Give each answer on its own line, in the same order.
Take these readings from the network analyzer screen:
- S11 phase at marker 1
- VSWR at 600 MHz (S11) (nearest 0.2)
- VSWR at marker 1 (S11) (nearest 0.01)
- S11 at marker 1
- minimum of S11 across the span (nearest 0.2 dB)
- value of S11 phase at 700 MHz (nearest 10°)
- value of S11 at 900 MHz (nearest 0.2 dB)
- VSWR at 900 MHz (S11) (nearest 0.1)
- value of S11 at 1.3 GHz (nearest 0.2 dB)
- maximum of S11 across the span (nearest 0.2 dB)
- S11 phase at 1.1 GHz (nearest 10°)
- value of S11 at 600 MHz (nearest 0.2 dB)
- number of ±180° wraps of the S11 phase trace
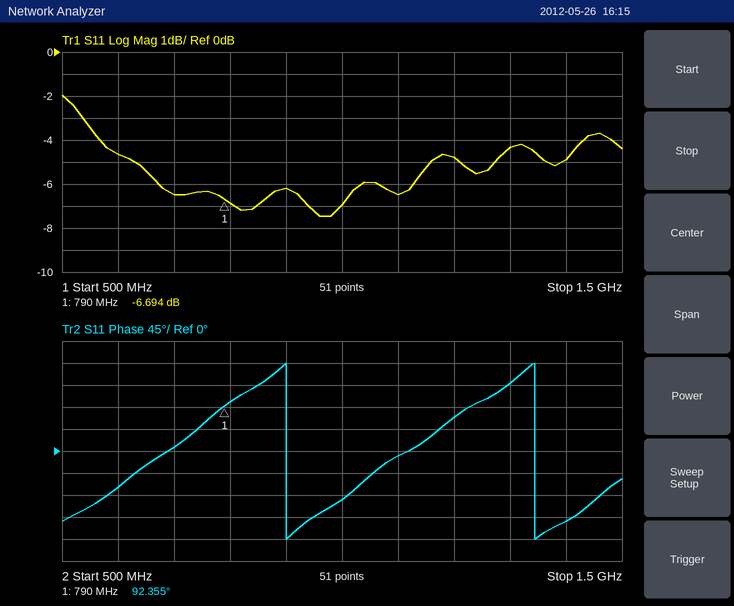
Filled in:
92.355°
3.8
2.72
-6.694 dB
-7.4 dB
10°
-6.2 dB
2.9
-4.4 dB
-2.0 dB
-10°
-4.6 dB
2
